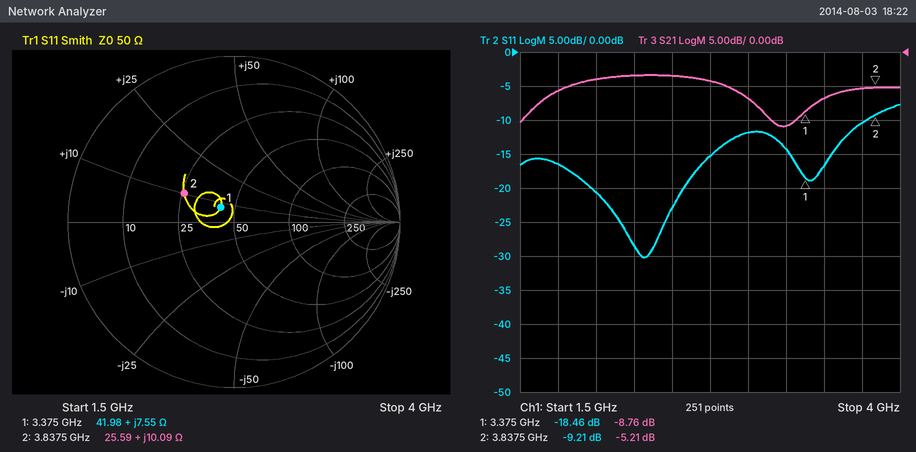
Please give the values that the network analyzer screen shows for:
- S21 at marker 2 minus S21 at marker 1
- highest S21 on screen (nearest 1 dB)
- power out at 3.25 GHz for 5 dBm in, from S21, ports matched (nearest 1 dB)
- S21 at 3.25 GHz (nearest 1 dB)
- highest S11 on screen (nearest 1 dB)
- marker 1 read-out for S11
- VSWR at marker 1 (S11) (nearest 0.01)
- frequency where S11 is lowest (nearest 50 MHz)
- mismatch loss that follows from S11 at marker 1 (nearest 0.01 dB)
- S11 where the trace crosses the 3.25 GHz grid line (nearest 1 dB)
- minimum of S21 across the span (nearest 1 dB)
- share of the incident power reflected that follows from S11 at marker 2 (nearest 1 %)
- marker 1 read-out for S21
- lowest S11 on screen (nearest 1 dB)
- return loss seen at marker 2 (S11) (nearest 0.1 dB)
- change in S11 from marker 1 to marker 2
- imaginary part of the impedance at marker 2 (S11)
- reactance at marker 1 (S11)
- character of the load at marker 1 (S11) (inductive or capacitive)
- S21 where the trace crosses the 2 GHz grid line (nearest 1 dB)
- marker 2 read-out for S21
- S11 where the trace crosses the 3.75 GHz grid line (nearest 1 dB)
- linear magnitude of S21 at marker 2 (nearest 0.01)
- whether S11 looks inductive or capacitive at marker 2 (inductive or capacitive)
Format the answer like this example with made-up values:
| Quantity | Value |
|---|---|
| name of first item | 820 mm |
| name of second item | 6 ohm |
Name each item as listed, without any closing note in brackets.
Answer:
| Quantity | Value |
|---|---|
| S21 at marker 2 minus S21 at marker 1 | 3.55 dB |
| highest S21 on screen | -3 dB |
| power out at 3.25 GHz for 5 dBm in, from S21, ports matched | -6 dBm |
| S21 at 3.25 GHz | -11 dB |
| highest S11 on screen | -8 dB |
| marker 1 read-out for S11 | -18.46 dB |
| VSWR at marker 1 (S11) | 1.27 |
| frequency where S11 is lowest | 2.30 GHz |
| mismatch loss that follows from S11 at marker 1 | 0.06 dB |
| S11 where the trace crosses the 3.25 GHz grid line | -14 dB |
| minimum of S21 across the span | -11 dB |
| share of the incident power reflected that follows from S11 at marker 2 | 12 % |
| marker 1 read-out for S21 | -8.76 dB |
| lowest S11 on screen | -30 dB |
| return loss seen at marker 2 (S11) | 9.2 dB |
| change in S11 from marker 1 to marker 2 | 9.25 dB |
| imaginary part of the impedance at marker 2 | +10.09 Ω |
| reactance at marker 1 | +7.55 Ω |
| character of the load at marker 1 (S11) | inductive |
| S21 where the trace crosses the 2 GHz grid line | -4 dB |
| marker 2 read-out for S21 | -5.21 dB |
| S11 where the trace crosses the 3.75 GHz grid line | -10 dB |
| linear magnitude of S21 at marker 2 | 0.55 |
| whether S11 looks inductive or capacitive at marker 2 | inductive |
